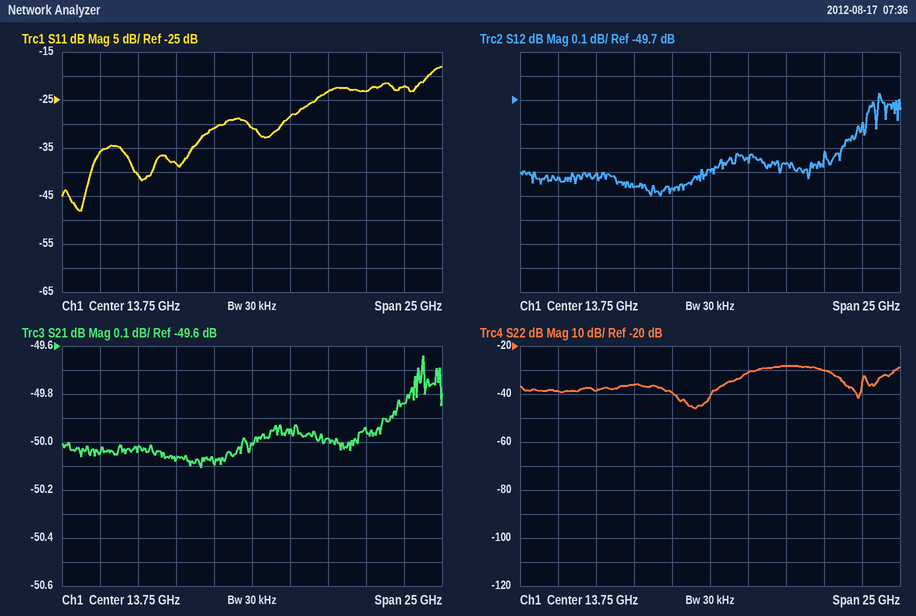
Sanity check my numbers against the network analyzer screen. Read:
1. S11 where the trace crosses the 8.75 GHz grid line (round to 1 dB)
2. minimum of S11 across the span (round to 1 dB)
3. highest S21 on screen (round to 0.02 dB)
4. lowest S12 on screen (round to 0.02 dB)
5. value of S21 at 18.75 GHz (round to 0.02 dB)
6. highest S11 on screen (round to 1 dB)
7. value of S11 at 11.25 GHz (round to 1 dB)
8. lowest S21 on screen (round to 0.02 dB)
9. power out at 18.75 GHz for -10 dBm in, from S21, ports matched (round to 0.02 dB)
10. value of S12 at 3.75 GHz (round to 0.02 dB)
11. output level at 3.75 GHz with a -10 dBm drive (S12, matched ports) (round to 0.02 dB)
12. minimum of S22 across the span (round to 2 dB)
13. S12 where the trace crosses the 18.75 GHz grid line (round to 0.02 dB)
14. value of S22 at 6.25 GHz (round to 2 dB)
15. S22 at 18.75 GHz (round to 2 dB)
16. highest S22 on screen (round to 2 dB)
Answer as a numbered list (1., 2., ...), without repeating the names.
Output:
1. -38 dB
2. -48 dB
3. -49.64 dB
4. -50.10 dB
5. -49.98 dB
6. -18 dB
7. -31 dB
8. -50.10 dB
9. -59.98 dBm
10. -50.02 dB
11. -60.02 dBm
12. -46 dB
13. -49.96 dB
14. -38 dB
15. -28 dB
16. -28 dB
